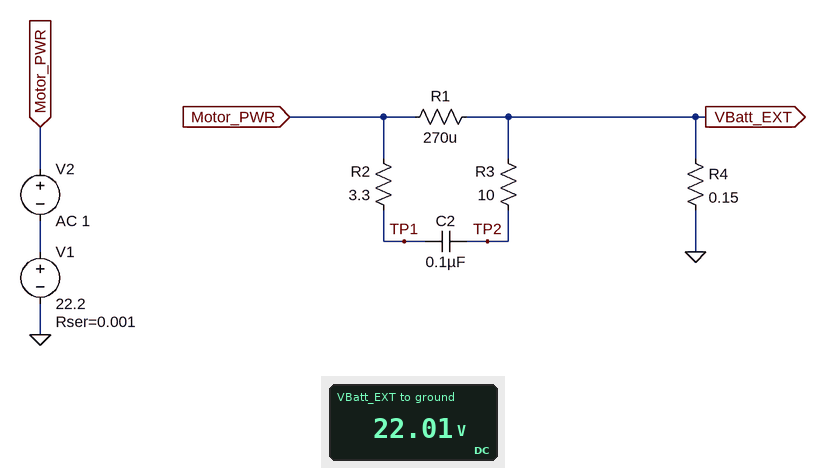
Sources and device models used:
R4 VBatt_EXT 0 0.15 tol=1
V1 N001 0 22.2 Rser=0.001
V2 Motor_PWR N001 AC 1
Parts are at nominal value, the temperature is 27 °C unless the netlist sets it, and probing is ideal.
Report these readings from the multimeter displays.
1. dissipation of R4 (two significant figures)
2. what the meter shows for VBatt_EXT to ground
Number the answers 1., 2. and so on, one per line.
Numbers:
1. 3.2 kW
2. 22.01 V
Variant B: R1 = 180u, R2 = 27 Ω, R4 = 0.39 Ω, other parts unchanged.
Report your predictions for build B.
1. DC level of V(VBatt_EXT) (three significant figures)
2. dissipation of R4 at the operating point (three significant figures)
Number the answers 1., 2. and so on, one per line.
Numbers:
1. 22.1 V
2. 1.26 kW
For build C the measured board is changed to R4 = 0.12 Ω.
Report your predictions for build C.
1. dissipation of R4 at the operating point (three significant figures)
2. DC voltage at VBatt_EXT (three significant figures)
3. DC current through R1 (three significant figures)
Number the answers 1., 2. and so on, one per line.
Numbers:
1. 4.02 kW
2. 22.0 V
3. 183 A
